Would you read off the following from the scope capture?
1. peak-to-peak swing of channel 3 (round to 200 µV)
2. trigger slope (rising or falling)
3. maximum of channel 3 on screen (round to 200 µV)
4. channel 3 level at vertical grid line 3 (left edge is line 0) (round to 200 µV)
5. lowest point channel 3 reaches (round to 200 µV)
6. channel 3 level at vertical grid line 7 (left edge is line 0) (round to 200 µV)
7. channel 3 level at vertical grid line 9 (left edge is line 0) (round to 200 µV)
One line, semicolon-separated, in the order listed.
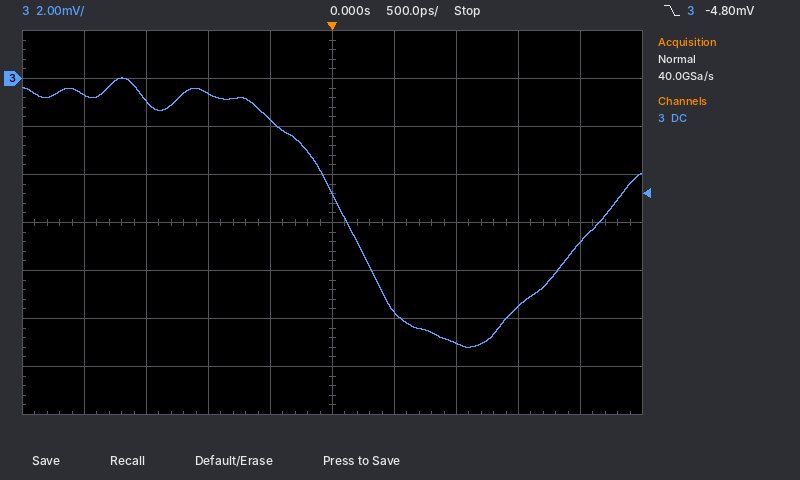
11.2 mV; falling; 0.0 mV; -600 µV; -11.2 mV; -11.0 mV; -6.8 mV
